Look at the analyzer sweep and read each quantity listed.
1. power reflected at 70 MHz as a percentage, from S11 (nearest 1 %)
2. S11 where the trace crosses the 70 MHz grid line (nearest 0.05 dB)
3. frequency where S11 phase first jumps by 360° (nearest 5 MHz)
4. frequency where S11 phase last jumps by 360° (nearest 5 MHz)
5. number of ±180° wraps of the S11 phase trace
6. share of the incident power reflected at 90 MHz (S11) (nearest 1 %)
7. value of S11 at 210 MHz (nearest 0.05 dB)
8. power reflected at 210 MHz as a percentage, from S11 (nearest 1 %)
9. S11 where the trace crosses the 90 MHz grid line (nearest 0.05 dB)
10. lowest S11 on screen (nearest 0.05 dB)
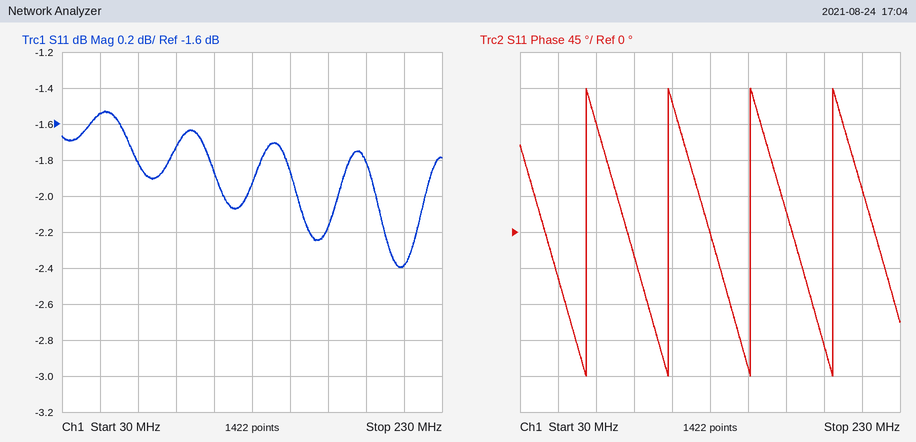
66 %
-1.80 dB
65 MHz
195 MHz
4
67 %
-2.40 dB
58 %
-1.75 dB
-2.40 dB
